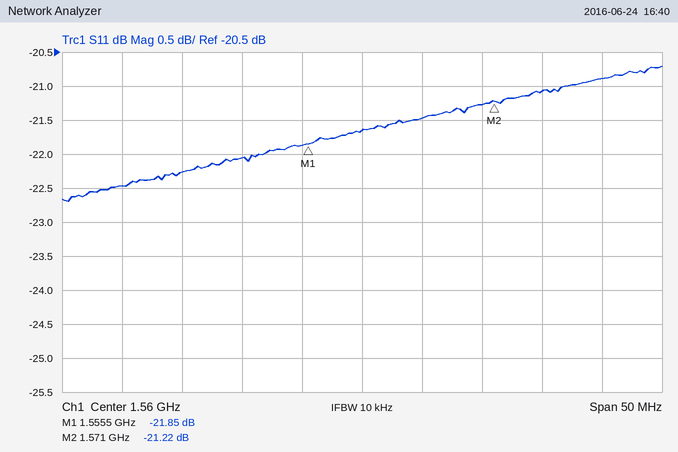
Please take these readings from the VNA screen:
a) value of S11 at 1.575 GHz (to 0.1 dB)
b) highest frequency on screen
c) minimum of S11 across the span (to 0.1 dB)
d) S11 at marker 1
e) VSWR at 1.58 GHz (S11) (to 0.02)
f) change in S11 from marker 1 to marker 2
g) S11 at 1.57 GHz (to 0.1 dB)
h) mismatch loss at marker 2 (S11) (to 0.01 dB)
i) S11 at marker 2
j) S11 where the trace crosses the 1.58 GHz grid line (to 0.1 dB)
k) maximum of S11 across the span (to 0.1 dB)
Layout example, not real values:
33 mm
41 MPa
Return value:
-21.1 dB
1.585 GHz
-22.7 dB
-21.85 dB
1.20
0.63 dB
-21.3 dB
0.03 dB
-21.22 dB
-20.9 dB
-20.7 dB
